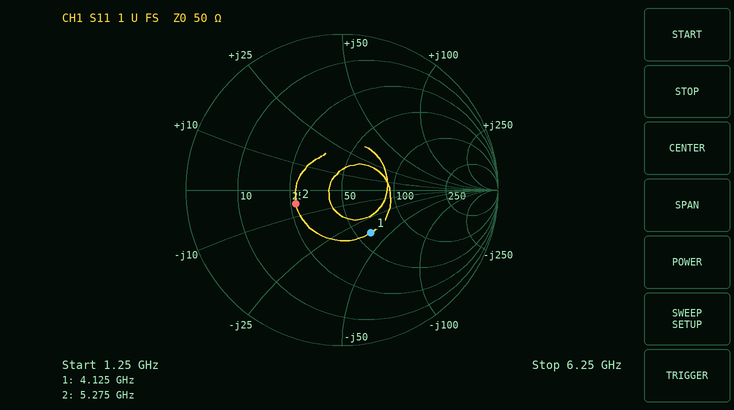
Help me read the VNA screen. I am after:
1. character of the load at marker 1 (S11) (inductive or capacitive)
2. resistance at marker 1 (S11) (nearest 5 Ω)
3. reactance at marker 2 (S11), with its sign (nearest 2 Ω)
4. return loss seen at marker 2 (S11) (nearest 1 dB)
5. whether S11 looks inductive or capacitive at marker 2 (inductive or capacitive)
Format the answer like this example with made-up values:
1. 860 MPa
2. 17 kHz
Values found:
1. capacitive
2. 60 Ω
3. -6 Ω
4. 10 dB
5. capacitive
